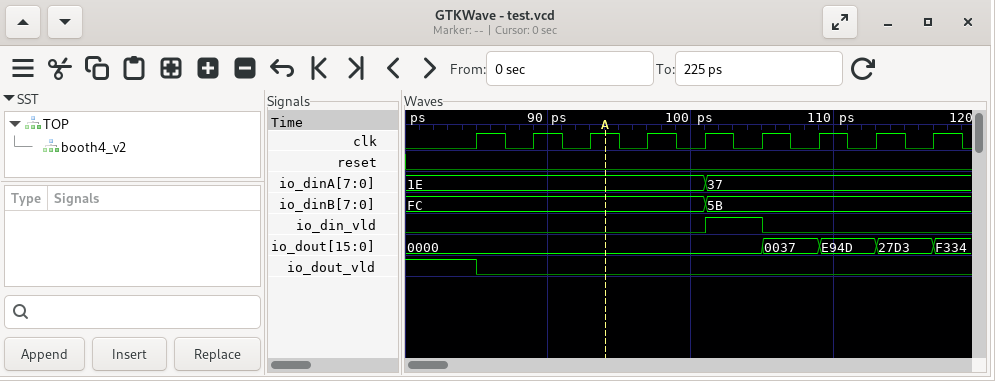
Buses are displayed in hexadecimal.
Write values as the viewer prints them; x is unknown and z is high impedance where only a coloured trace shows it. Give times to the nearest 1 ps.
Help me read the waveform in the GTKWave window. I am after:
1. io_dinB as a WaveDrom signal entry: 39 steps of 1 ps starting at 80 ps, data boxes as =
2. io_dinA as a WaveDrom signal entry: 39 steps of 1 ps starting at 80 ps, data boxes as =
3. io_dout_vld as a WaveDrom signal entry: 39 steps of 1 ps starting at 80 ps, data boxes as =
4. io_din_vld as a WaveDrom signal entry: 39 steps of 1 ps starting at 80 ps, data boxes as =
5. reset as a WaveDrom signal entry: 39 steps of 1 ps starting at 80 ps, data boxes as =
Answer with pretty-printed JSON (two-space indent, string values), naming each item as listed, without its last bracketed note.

{
  "io_dinB as a WaveDrom signal entry: 39 steps of 1 ps starting at 80 ps, data boxes as =": "{name: 'io_dinB', wave: '=....................=.................', data: 'FC 5B'}",
  "io_dinA as a WaveDrom signal entry: 39 steps of 1 ps starting at 80 ps, data boxes as =": "{name: 'io_dinA', wave: '=....................=.................', data: '1E 37'}",
  "io_dout_vld as a WaveDrom signal entry: 39 steps of 1 ps starting at 80 ps, data boxes as =": "{name: 'io_dout_vld', wave: '1....0.................................'}",
  "io_din_vld as a WaveDrom signal entry: 39 steps of 1 ps starting at 80 ps, data boxes as =": "{name: 'io_din_vld', wave: '0....................1...0.............'}",
  "reset as a WaveDrom signal entry: 39 steps of 1 ps starting at 80 ps, data boxes as =": "{name: 'reset', wave: '0......................................'}"
}
